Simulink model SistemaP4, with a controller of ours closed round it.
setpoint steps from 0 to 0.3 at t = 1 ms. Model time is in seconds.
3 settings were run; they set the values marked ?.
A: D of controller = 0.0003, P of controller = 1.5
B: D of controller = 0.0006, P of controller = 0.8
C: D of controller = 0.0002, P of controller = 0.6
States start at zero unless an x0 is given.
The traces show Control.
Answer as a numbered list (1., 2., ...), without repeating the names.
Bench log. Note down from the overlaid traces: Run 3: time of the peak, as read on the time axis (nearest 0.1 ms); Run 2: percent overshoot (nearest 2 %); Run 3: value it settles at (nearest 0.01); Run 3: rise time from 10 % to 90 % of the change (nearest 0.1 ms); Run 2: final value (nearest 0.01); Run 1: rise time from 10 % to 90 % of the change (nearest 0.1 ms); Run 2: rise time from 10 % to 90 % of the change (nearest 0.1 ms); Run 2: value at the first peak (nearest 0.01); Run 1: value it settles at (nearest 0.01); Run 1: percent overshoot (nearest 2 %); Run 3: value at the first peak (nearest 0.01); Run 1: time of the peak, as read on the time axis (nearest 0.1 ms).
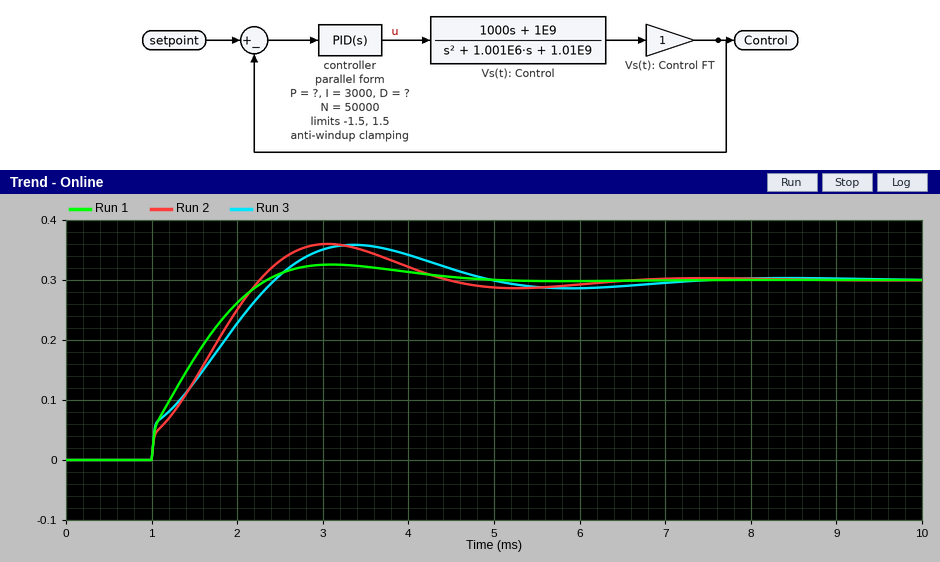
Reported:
1. 3.4 ms
2. 20 %
3. 0.30
4. 1.2 ms
5. 0.30
6. 1.0 ms
7. 1.1 ms
8. 0.36
9. 0.30
10. 8 %
11. 0.36
12. 3.1 ms
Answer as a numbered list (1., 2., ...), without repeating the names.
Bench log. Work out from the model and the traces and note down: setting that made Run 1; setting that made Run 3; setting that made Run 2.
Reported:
1. A
2. B
3. C
